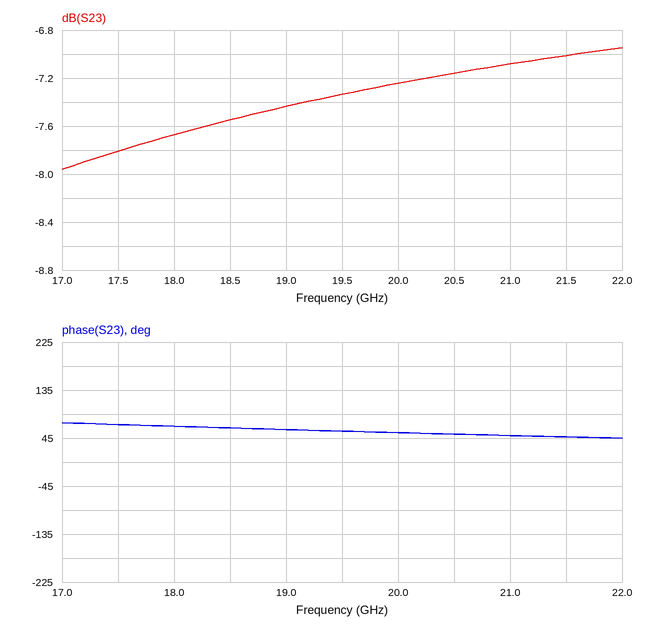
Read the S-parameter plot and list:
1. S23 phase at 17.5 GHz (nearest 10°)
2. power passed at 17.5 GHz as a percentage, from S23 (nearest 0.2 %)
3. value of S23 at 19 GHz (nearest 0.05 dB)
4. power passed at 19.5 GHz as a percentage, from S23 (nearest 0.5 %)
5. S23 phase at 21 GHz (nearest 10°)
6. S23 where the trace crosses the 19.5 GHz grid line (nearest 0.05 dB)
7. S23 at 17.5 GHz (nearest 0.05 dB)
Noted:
70°
16.6 %
-7.45 dB
18.5 %
50°
-7.35 dB
-7.80 dB
